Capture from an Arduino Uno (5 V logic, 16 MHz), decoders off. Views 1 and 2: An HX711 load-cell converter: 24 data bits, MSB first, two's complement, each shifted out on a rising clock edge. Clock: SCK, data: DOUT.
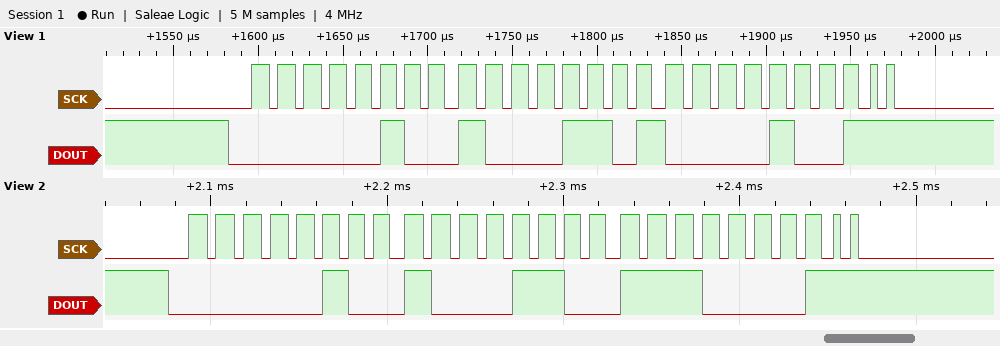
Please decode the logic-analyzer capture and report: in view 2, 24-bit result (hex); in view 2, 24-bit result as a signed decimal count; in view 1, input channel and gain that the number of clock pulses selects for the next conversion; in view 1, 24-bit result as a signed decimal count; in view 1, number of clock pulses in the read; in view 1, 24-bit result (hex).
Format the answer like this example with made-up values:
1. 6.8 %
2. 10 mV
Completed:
1. 0x048CE1
2. 298209
3. channel B, gain 32
4. 298249
5. 26
6. 0x048D09
